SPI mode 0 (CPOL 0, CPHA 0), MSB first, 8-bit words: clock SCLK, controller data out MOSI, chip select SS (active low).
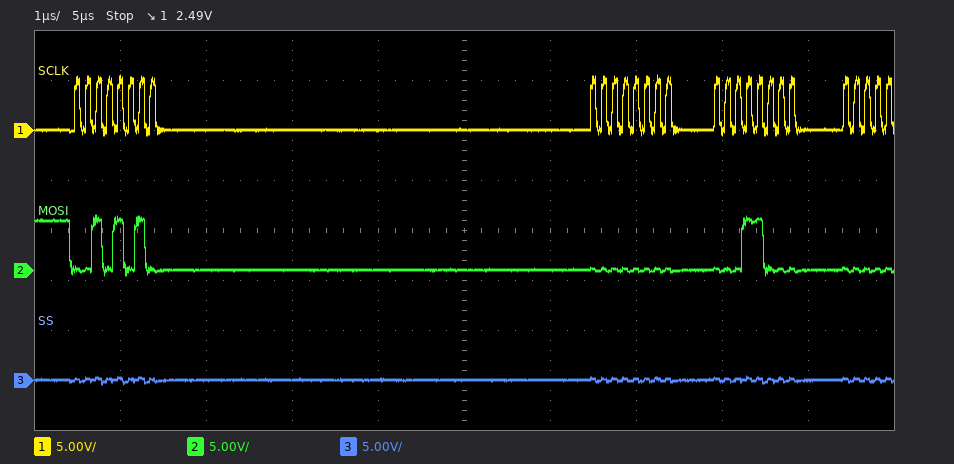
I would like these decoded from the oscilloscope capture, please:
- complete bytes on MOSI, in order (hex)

0x2A 0x00 0x18
